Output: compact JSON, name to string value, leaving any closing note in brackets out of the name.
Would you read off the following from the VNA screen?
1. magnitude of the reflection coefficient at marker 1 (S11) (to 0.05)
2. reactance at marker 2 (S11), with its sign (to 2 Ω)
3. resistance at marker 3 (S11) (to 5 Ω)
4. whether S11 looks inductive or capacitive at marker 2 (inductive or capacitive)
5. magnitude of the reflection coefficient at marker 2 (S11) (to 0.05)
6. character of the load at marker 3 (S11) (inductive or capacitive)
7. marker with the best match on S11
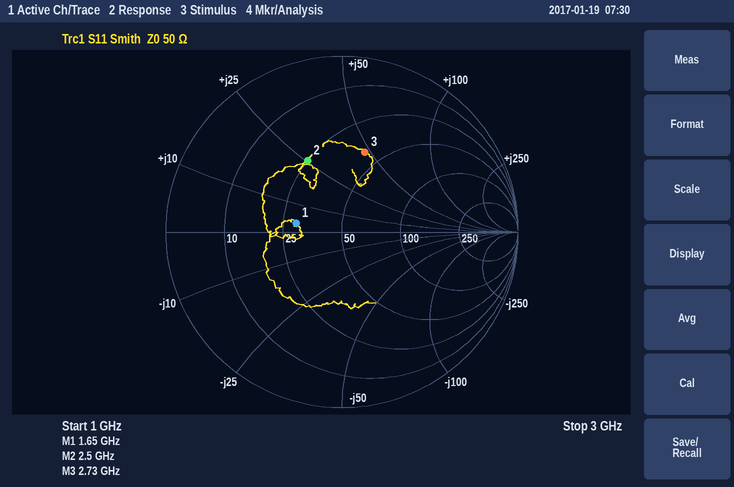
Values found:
{"magnitude of the reflection coefficient at marker 1 (S11)": "0.25", "reactance at marker 2 (S11), with its sign": "+26 Ω", "resistance at marker 3 (S11)": "40 Ω", "whether S11 looks inductive or capacitive at marker 2": "inductive", "magnitude of the reflection coefficient at marker 2 (S11)": "0.45", "character of the load at marker 3 (S11)": "inductive", "marker with the best match on S11": "marker 1"}
